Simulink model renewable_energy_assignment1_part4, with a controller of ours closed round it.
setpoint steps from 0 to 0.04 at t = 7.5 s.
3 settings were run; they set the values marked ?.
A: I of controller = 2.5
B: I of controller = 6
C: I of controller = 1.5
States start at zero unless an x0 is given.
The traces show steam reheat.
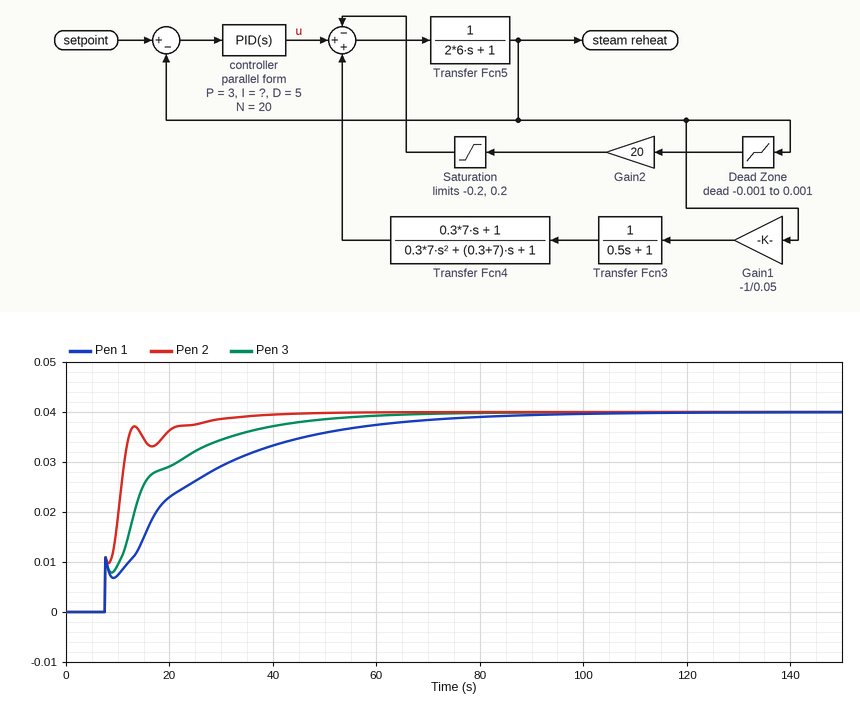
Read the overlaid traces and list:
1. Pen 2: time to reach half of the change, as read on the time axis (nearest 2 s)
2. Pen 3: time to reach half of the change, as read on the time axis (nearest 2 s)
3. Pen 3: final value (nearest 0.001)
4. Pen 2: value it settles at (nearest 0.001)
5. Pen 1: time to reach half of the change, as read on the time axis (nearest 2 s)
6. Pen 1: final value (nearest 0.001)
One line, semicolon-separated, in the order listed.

10 s; 14 s; 0.040; 0.040; 18 s; 0.040
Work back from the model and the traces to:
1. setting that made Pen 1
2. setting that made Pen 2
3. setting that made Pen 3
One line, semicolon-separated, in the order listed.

C; B; A
